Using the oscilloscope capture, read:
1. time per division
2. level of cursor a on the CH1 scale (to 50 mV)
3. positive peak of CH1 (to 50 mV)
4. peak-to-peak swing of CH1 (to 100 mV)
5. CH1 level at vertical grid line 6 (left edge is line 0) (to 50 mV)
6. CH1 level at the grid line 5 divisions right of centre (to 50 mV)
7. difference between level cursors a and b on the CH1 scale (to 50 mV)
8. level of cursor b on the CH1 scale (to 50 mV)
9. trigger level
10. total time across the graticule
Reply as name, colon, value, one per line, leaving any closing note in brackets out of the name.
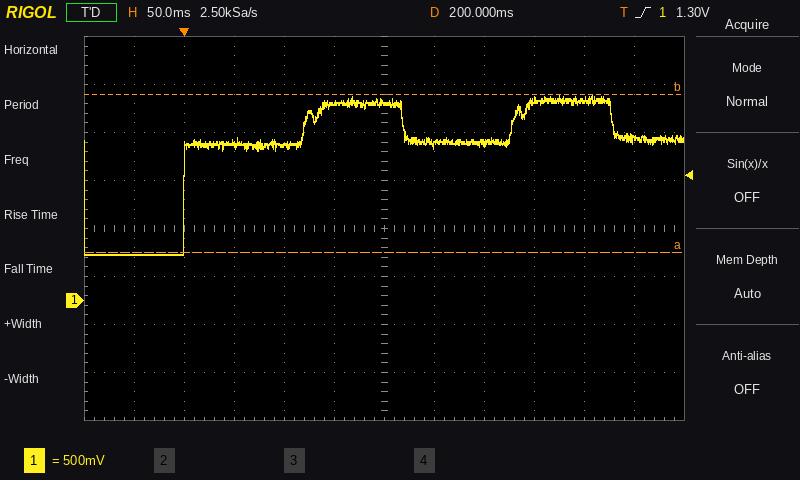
time per division: 50 ms
level of cursor a on the CH1 scale: 500 mV
positive peak of CH1: 2.15 V
peak-to-peak swing of CH1: 1.70 V
CH1 level at vertical grid line 6 (left edge is line 0): 2.05 V
CH1 level at the grid line 5 divisions right of centre: 1.70 V
difference between level cursors a and b on the CH1 scale: 1.65 V
level of cursor b on the CH1 scale: 2.15 V
trigger level: 1.30 V
total time across the graticule: 600 ms
